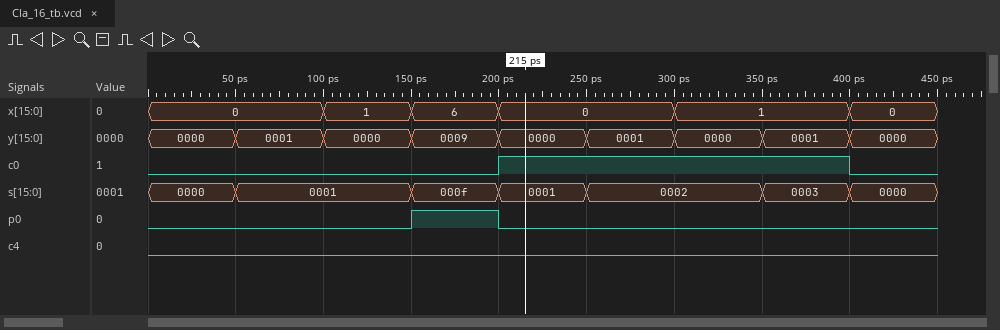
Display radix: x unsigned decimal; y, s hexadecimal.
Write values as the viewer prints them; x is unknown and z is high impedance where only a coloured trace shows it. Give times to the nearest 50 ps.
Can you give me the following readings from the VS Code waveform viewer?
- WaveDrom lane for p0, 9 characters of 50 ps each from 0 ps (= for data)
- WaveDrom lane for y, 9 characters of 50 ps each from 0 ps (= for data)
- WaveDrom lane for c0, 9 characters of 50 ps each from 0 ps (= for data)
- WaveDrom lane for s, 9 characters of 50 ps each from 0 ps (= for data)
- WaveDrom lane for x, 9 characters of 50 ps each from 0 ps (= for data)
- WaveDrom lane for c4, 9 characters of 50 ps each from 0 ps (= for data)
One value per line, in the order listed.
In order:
{name: 'p0', wave: '0..10....'}
{name: 'y', wave: '=========', data: '0000 0001 0000 0009 0000 0001 0000 0001 0000'}
{name: 'c0', wave: '0...1...0'}
{name: 's', wave: '==.===.==', data: '0000 0001 000f 0001 0002 0003 0000'}
{name: 'x', wave: '=.===.=.=', data: '0 1 6 0 1 0'}
{name: 'c4', wave: '0........'}
